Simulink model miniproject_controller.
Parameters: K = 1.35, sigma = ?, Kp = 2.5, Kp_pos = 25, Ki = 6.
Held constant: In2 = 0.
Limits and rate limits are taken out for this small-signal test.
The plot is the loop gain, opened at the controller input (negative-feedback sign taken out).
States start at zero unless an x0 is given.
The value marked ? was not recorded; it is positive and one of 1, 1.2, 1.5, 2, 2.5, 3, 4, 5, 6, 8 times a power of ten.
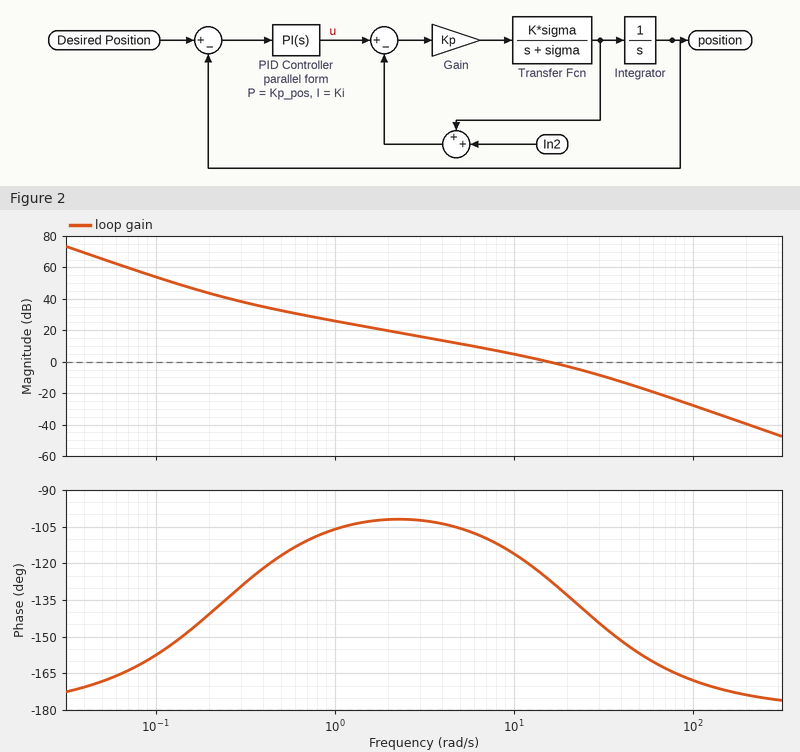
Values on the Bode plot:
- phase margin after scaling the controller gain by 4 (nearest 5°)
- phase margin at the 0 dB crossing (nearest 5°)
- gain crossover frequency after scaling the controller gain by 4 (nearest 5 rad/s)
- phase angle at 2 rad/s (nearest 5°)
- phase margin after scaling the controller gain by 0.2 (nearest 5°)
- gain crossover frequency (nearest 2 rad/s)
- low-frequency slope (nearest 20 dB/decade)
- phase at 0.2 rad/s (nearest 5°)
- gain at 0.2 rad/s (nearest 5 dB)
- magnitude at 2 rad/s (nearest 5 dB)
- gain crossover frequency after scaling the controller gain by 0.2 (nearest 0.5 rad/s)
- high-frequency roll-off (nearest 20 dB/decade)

30°
55°
40 rad/s
-100°
75°
16 rad/s
-40 dB/decade
-140°
45 dB
20 dB
4.0 rad/s
-40 dB/decade
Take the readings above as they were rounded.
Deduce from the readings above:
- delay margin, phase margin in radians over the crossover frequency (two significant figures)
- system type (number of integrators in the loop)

0.060 s
2
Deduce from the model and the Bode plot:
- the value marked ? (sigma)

5
